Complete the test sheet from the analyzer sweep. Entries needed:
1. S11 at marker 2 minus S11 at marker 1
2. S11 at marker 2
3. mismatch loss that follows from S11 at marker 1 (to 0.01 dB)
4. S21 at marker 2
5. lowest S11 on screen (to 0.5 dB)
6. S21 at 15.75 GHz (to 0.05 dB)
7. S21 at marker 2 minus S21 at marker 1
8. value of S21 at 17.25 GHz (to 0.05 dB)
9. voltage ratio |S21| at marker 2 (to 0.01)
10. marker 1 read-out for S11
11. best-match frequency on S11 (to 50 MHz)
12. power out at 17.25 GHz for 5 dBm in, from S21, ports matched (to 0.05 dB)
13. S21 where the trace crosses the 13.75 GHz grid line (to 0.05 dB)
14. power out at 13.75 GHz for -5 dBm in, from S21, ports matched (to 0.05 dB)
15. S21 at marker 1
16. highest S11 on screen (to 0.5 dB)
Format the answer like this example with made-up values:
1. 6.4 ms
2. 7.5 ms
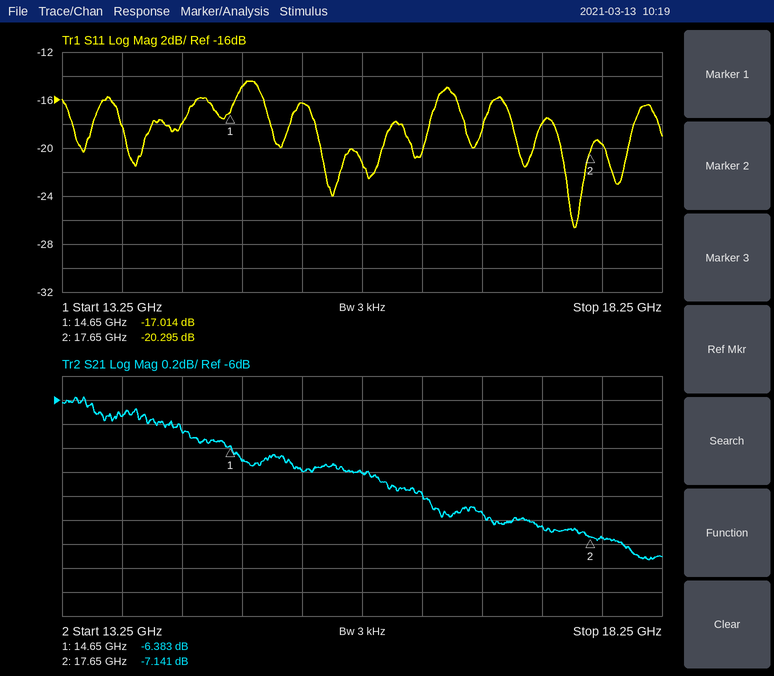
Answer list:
1. -3.281 dB
2. -20.295 dB
3. 0.09 dB
4. -7.141 dB
5. -26.5 dB
6. -6.60 dB
7. -0.758 dB
8. -7.05 dB
9. 0.44
10. -17.014 dB
11. 17.50 GHz
12. -2.05 dBm
13. -6.15 dB
14. -11.15 dBm
15. -6.383 dB
16. -14.5 dB
